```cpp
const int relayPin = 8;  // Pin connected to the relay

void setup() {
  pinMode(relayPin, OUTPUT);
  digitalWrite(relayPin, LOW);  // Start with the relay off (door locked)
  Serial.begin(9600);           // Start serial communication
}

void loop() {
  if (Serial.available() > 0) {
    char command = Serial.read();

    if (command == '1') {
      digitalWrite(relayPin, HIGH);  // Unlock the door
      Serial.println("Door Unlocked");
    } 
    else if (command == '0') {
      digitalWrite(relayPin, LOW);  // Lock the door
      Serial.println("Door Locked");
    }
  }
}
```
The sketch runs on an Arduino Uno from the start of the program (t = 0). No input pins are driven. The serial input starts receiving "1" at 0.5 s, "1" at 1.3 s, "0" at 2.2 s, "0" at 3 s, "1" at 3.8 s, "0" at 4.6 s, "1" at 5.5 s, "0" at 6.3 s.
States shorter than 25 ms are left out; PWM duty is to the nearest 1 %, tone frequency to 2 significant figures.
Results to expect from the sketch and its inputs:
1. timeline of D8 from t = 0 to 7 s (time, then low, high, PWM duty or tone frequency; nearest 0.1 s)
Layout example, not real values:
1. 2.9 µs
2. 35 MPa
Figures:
1. 0 s low; 0.5 s high; 2.2 s low; 3.8 s high; 4.6 s low; 5.5 s high; 6.3 s low
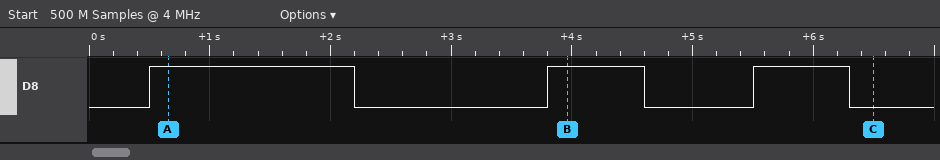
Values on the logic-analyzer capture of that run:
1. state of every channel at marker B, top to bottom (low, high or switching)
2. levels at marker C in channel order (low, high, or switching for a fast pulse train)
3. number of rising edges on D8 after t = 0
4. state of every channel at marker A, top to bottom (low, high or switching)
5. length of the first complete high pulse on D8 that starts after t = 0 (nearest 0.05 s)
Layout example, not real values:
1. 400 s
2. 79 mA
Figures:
1. D8 high
2. D8 low
3. 3
4. D8 high
5. 1.70 s
